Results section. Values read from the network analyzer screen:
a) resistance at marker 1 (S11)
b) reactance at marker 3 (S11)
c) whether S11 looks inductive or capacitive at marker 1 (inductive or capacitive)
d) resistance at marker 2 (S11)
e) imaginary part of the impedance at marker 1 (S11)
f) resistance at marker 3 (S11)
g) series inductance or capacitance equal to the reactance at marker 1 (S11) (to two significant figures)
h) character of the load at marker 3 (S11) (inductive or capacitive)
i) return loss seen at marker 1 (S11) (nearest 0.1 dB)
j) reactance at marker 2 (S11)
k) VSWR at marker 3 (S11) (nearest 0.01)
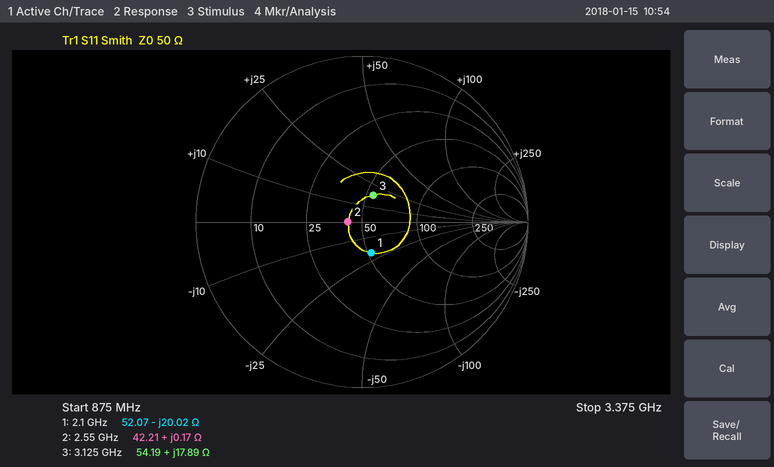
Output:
52.07 Ω
+17.89 Ω
capacitive
42.21 Ω
-20.02 Ω
54.19 Ω
3.8 pF
inductive
14.3 dB
+0.17 Ω
1.42
